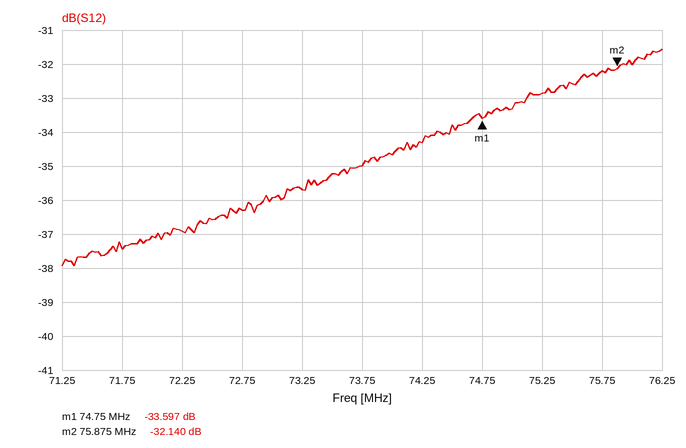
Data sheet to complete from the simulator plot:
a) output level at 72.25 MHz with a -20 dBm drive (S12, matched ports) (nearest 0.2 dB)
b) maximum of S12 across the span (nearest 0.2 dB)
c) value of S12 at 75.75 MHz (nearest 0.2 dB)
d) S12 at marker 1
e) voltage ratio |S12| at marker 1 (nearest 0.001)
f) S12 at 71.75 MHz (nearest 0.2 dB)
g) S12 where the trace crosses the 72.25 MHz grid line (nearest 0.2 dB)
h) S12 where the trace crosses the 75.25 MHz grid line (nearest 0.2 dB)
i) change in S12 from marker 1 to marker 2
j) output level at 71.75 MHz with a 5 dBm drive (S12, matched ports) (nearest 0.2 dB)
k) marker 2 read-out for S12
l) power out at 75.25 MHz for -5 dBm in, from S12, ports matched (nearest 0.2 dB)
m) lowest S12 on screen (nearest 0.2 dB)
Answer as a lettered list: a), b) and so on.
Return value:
a) -57.0 dBm
b) -31.6 dB
c) -32.2 dB
d) -33.597 dB
e) 0.021
f) -37.4 dB
g) -37.0 dB
h) -32.8 dB
i) 1.457 dB
j) -32.4 dBm
k) -32.140 dB
l) -37.8 dBm
m) -38.0 dB
